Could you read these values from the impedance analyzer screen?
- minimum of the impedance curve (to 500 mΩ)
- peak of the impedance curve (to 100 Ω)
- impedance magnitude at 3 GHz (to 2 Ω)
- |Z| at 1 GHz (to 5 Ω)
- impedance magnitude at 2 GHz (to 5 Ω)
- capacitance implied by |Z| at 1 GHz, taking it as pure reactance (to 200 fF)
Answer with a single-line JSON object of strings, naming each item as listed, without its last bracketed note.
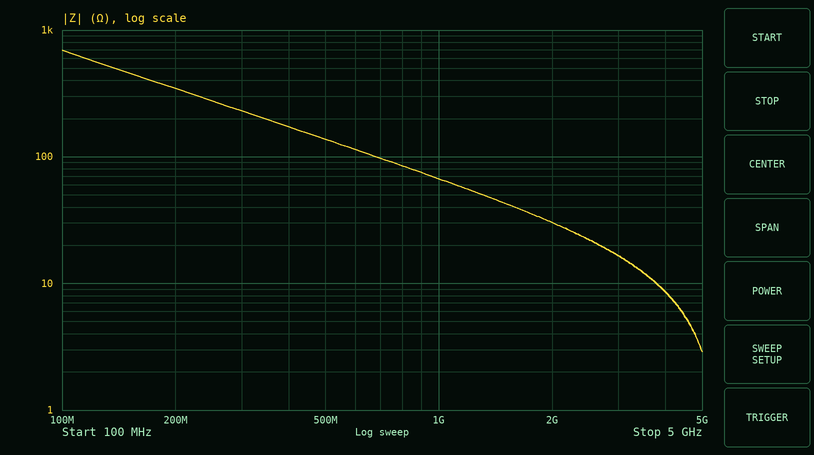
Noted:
{"minimum of the impedance curve": "3.0 Ω", "peak of the impedance curve": "700 Ω", "impedance magnitude at 3 GHz": "16 Ω", "|Z| at 1 GHz": "65 Ω", "impedance magnitude at 2 GHz": "30 Ω", "capacitance implied by |Z| at 1 GHz, taking it as pure reactance": "2.4 pF"}
